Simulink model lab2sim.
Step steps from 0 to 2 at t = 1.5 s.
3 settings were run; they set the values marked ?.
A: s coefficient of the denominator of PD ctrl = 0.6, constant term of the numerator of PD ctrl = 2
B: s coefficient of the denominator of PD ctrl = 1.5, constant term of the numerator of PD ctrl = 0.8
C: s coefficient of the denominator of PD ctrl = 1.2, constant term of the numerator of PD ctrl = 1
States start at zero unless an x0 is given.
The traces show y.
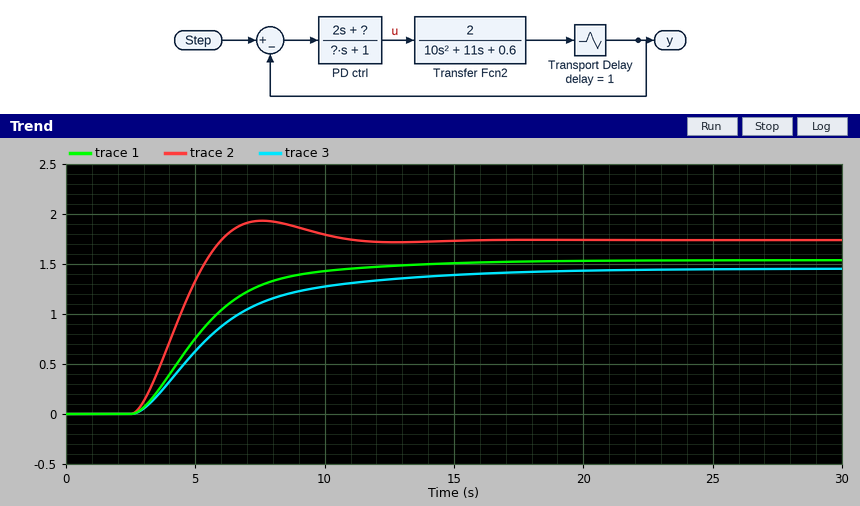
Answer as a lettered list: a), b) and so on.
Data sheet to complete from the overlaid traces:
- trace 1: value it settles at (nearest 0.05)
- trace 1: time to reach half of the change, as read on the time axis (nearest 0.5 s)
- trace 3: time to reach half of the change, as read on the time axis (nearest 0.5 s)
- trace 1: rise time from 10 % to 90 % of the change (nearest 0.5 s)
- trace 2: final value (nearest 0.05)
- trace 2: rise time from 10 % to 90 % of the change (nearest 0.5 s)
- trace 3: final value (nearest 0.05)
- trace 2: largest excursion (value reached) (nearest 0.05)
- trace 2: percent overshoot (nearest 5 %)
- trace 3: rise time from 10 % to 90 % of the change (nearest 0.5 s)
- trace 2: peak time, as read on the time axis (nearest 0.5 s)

a) 1.55
b) 5.0 s
c) 5.5 s
d) 5.5 s
e) 1.75
f) 2.5 s
g) 1.45
h) 1.95
i) 10 %
j) 7.5 s
k) 7.5 s
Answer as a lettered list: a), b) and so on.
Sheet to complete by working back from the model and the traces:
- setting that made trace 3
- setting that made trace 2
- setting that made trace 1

a) B
b) A
c) C
